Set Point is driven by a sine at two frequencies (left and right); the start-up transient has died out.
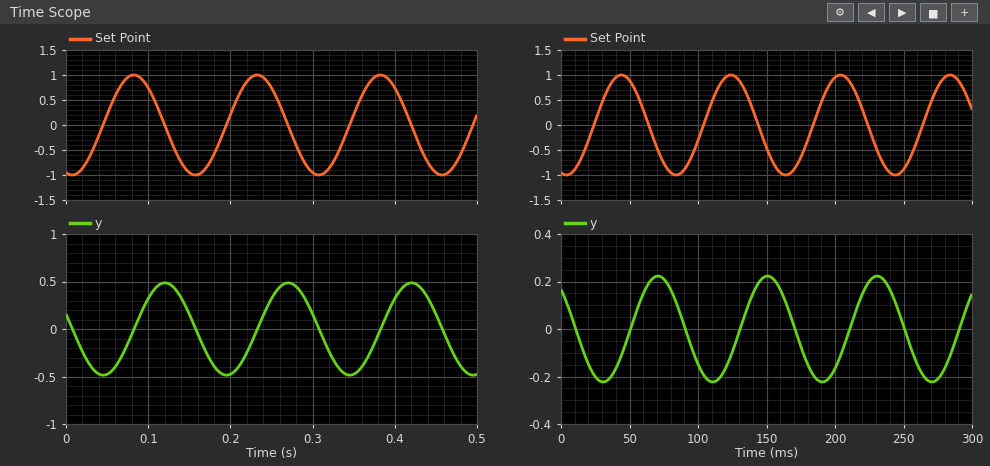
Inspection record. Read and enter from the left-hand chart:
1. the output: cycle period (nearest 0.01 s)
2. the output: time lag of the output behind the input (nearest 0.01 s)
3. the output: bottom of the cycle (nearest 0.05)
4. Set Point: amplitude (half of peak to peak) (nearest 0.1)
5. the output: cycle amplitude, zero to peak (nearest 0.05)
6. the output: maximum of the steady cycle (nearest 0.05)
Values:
0.15 s
0.04 s
-0.50
1.0
0.50
0.50
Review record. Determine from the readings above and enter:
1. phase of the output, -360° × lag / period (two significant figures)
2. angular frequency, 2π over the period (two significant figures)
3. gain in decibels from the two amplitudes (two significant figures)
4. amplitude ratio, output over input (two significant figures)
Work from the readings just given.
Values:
-96°
42 rad/s
-6.0 dB
0.50
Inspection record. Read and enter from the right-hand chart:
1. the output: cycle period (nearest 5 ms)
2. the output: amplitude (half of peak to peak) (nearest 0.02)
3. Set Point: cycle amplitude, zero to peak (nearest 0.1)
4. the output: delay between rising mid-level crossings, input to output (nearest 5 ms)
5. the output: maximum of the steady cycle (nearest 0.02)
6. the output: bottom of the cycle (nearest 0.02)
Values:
80 ms
0.22
1.0
25 ms
0.22
-0.22
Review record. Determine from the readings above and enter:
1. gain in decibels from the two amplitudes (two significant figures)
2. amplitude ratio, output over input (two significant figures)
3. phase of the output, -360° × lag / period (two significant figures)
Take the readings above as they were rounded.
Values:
-13 dB
0.22
-110°
